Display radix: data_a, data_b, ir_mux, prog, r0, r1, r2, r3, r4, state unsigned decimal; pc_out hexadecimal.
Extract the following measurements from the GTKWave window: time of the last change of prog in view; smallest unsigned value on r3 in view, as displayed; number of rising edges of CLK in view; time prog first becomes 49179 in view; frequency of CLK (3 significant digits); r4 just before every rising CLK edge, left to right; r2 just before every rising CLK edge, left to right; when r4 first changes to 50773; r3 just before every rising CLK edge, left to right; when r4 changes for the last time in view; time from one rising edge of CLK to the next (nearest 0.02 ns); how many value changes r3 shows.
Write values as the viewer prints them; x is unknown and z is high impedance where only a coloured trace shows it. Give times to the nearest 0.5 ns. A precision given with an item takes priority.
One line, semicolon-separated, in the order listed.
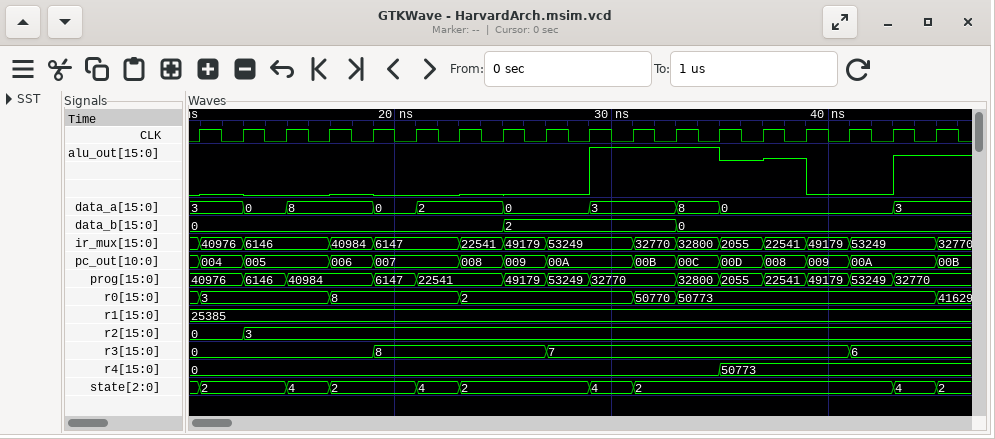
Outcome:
43 ns; 0; 18; 25 ns; 500 MHz; 0, 0, 0, 0, 0, 0, 0, 0, 0, 0, 0, 0, 0, 50773, 50773, 50773, 50773, 50773; 0, 0, 3, 3, 3, 3, 3, 3, 3, 3, 3, 3, 3, 3, 3, 3, 3, 3; 35 ns; 0, 0, 0, 0, 0, 8, 8, 8, 8, 7, 7, 7, 7, 7, 7, 7, 6, 6; 35 ns; 2 ns; 3
